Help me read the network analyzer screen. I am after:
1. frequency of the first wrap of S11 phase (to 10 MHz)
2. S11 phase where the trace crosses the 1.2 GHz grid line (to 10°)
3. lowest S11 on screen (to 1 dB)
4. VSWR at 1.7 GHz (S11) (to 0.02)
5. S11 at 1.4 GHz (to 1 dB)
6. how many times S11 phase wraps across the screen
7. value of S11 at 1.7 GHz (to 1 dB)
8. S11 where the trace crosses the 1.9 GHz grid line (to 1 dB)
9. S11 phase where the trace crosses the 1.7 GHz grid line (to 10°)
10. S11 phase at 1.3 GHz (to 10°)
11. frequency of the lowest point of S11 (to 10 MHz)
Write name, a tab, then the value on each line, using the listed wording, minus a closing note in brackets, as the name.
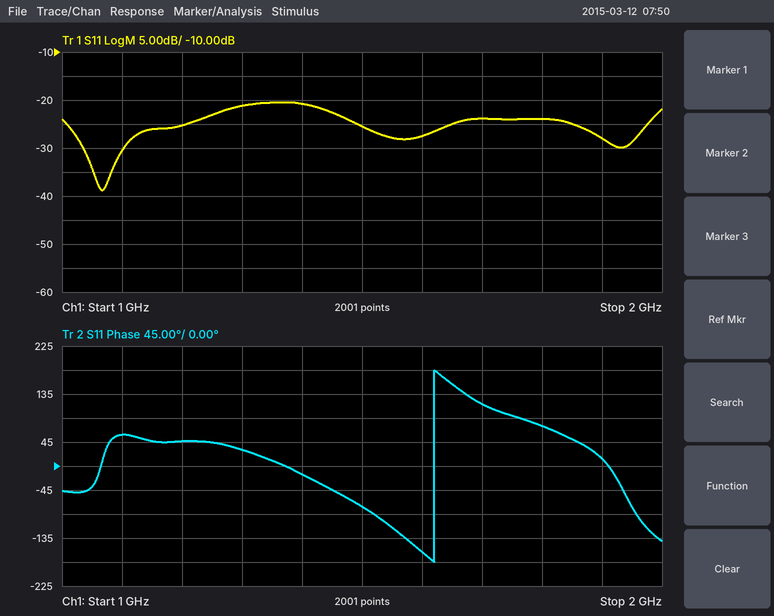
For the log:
frequency of the first wrap of S11 phase	1.62 GHz
S11 phase where the trace crosses the 1.2 GHz grid line	50°
lowest S11 on screen	-39 dB
VSWR at 1.7 GHz (S11)	1.14
S11 at 1.4 GHz	-21 dB
how many times S11 phase wraps across the screen	1
value of S11 at 1.7 GHz	-24 dB
S11 where the trace crosses the 1.9 GHz grid line	-28 dB
S11 phase where the trace crosses the 1.7 GHz grid line	120°
S11 phase at 1.3 GHz	30°
frequency of the lowest point of S11	1.07 GHz
